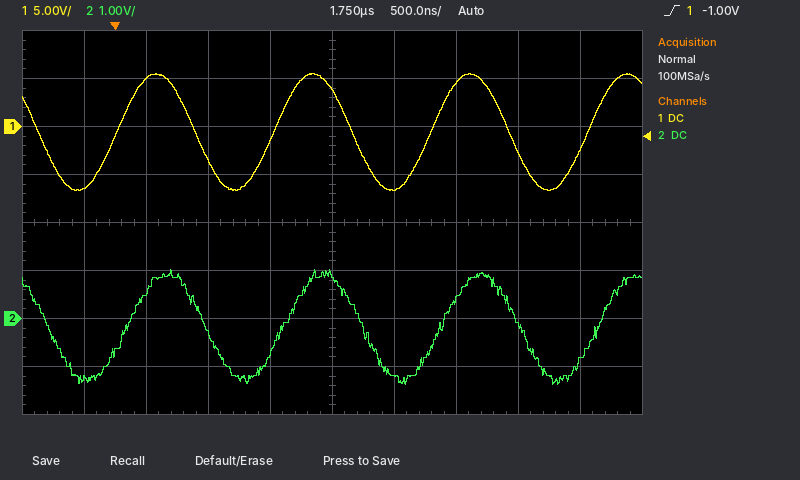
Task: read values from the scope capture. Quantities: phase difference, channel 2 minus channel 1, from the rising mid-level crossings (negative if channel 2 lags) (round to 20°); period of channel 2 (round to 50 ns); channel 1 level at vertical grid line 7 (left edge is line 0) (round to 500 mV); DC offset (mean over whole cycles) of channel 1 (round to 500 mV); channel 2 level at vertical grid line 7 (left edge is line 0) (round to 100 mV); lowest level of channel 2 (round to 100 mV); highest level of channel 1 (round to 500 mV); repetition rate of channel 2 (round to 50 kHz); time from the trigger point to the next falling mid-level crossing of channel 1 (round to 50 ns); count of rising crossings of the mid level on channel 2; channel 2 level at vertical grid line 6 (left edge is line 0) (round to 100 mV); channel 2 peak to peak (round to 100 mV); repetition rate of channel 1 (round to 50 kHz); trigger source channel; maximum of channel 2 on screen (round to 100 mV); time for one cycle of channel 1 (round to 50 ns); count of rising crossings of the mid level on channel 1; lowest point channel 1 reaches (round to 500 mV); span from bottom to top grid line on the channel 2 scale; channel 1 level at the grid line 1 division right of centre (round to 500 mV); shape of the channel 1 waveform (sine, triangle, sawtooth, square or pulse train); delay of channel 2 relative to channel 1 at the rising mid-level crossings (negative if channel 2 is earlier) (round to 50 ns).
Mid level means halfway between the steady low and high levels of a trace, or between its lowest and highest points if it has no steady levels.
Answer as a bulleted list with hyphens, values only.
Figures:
- -20°
- 1.25 µs
- 4.5 V
- -500 mV
- 400 mV
- -1.4 V
- 5.5 V
- 800 kHz
- 650 ns
- 4
- -1.2 V
- 2.4 V
- 800 kHz
- channel 1
- 1.0 V
- 1.25 µs
- 4
- -6.5 V
- 8 V
- -6.5 V
- sine
- +100 ns
